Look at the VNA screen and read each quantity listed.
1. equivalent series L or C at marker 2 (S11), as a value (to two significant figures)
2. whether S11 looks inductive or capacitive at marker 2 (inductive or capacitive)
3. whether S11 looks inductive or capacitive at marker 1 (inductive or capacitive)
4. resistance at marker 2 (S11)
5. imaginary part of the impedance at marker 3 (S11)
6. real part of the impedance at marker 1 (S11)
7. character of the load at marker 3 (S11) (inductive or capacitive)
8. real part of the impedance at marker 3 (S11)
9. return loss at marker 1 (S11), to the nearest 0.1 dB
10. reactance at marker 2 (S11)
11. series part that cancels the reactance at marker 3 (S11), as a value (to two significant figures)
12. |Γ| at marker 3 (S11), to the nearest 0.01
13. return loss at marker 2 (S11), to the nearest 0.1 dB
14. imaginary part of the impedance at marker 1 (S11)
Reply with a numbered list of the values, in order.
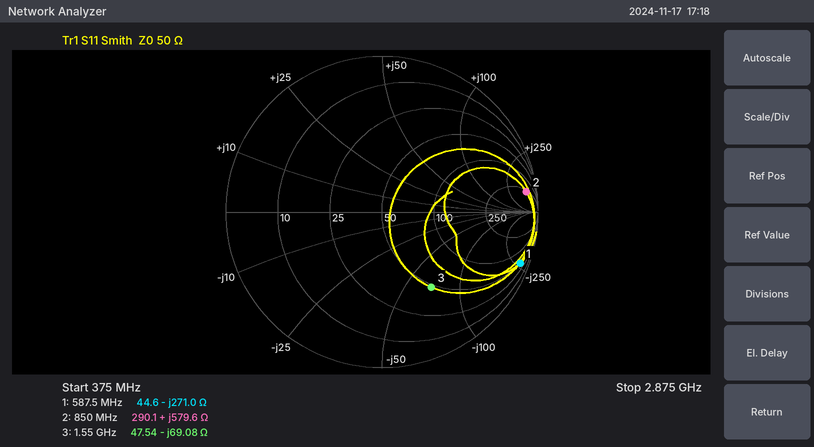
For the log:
1. 110 nH
2. inductive
3. capacitive
4. 290.1 Ω
5. -69.08 Ω
6. 44.6 Ω
7. capacitive
8. 47.54 Ω
9. 0.5 dB
10. +579.6 Ω
11. 7.1 nH
12. 0.58
13. 0.6 dB
14. -271.0 Ω
